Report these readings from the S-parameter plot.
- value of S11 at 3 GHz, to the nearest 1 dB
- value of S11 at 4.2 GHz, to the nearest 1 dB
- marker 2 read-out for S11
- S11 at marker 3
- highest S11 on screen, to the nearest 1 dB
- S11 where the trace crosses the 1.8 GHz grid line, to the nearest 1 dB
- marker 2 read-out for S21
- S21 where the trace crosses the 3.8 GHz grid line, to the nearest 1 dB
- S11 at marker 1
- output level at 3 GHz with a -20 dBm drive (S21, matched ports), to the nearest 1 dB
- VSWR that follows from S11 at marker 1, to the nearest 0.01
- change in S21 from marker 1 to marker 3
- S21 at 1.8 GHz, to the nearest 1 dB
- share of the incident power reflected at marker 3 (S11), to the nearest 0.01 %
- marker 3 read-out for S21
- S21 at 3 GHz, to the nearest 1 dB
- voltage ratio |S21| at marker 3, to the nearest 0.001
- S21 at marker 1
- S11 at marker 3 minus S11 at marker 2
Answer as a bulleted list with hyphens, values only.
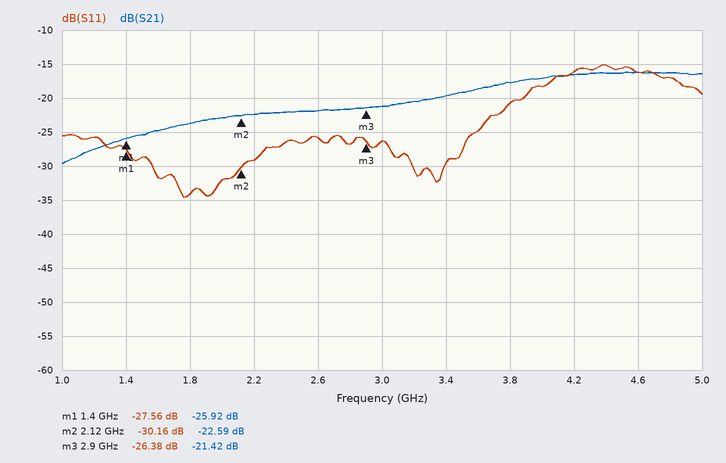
- -26 dB
- -16 dB
- -30.16 dB
- -26.38 dB
- -15 dB
- -34 dB
- -22.59 dB
- -18 dB
- -27.56 dB
- -41 dBm
- 1.09
- 4.50 dB
- -24 dB
- 0.23 %
- -21.42 dB
- -21 dB
- 0.085
- -25.92 dB
- 3.78 dB
